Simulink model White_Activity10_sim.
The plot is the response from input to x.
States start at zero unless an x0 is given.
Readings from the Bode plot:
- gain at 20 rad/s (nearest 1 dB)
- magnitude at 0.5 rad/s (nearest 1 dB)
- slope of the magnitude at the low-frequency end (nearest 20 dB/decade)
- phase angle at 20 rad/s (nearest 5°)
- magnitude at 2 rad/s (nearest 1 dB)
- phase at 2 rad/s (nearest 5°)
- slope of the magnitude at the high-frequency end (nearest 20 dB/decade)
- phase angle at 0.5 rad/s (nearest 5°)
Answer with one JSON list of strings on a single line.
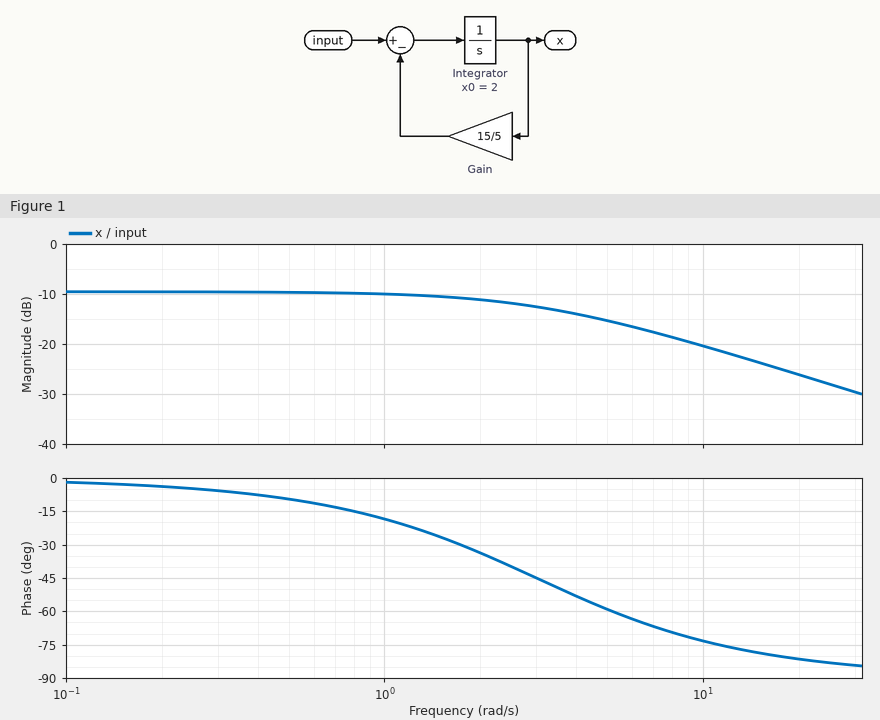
["-26 dB", "-10 dB", "0 dB/decade", "-80°", "-11 dB", "-35°", "-20 dB/decade", "-10°"]
